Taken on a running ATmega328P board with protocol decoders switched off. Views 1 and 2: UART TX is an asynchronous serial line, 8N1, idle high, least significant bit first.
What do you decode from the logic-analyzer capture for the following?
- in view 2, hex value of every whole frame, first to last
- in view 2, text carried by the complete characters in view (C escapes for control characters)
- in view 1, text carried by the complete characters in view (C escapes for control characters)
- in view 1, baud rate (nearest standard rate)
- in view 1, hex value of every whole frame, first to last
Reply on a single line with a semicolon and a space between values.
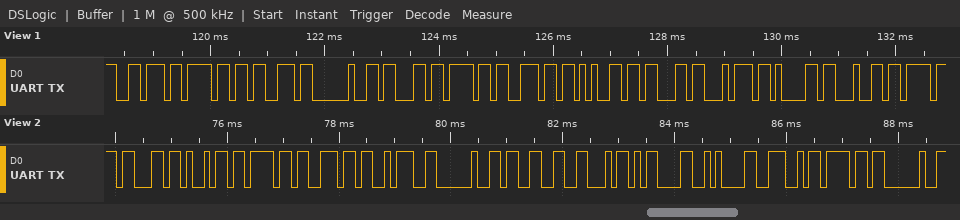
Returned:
63 69 6F 6E 3A 20 33 46 0D 0A 4E 6F 20; "cion: 3F\r\nNo "; "vos conectad"; 9600 baud; 76 6F 73 20 63 6F 6E 65 63 74 61 64
